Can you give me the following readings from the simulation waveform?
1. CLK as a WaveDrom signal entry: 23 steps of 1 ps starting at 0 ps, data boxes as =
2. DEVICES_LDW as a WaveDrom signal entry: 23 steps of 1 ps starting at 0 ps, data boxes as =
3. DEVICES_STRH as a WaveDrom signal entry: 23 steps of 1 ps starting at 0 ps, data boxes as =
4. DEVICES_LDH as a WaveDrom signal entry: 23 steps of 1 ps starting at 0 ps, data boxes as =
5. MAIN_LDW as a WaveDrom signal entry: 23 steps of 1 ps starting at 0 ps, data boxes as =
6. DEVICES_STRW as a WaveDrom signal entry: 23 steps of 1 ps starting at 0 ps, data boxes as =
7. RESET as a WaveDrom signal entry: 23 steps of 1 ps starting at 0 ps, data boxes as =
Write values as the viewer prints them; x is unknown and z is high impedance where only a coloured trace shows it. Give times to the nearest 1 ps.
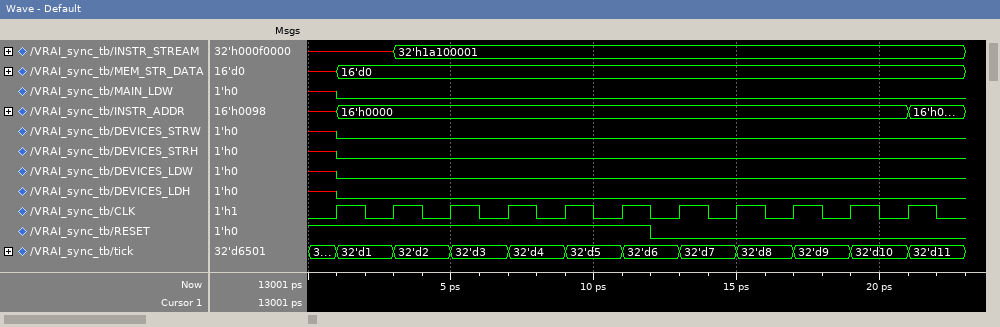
{name: 'CLK', wave: '01010101010101010101010'}
{name: 'DEVICES_LDW', wave: 'x0.....................'}
{name: 'DEVICES_STRH', wave: 'x0.....................'}
{name: 'DEVICES_LDH', wave: 'x0.....................'}
{name: 'MAIN_LDW', wave: 'x0.....................'}
{name: 'DEVICES_STRW', wave: 'x0.....................'}
{name: 'RESET', wave: '1...........0..........'}
